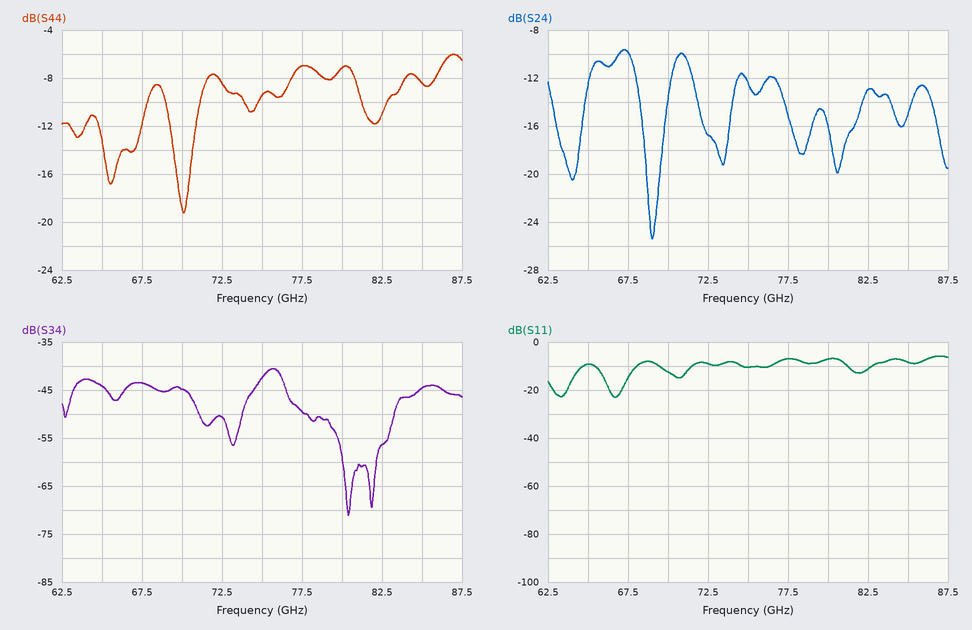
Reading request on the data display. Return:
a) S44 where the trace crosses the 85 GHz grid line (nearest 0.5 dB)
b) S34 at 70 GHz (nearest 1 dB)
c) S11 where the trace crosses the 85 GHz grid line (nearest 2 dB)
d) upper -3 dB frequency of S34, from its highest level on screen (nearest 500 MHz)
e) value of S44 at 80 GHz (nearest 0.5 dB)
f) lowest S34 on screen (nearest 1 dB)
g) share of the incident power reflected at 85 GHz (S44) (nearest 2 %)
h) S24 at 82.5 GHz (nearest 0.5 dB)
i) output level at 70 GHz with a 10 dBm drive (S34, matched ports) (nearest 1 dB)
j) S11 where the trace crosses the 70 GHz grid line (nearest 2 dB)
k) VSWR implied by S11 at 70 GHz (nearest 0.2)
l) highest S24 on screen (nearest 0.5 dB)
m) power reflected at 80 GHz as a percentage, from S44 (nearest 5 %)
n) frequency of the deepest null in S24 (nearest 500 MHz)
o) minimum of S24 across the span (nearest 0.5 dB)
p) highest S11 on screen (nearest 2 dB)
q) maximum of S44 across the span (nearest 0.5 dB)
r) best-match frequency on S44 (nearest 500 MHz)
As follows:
-8.5 dB
-45 dB
-8 dB
76.5 GHz
-7.0 dB
-71 dB
14 %
-13.0 dB
-35 dBm
-12 dB
1.6
-9.5 dB
20 %
69.0 GHz
-25.5 dB
-6 dB
-6.0 dB
70.0 GHz
